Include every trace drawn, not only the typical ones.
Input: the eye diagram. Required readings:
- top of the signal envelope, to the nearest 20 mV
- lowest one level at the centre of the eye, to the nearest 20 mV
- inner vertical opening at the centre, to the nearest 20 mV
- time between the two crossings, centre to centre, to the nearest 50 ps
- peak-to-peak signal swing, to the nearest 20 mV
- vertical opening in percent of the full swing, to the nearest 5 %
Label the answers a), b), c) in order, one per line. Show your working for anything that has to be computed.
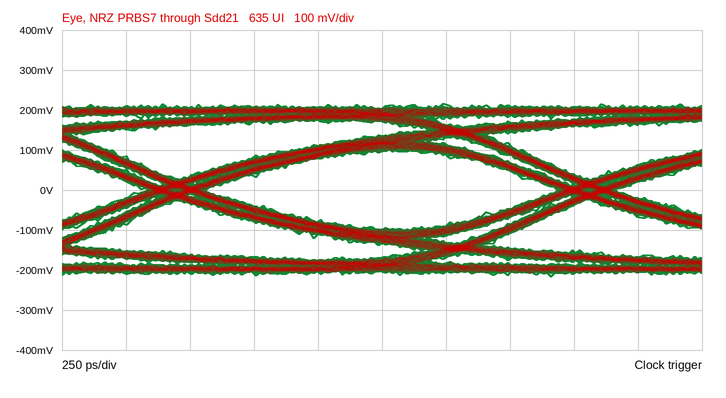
a) 220 mV
b) 100 mV
c) 200 mV
d) 1.60 ns
e) 440 mV
f) 200 mV / 440 mV ≈ 45 %
